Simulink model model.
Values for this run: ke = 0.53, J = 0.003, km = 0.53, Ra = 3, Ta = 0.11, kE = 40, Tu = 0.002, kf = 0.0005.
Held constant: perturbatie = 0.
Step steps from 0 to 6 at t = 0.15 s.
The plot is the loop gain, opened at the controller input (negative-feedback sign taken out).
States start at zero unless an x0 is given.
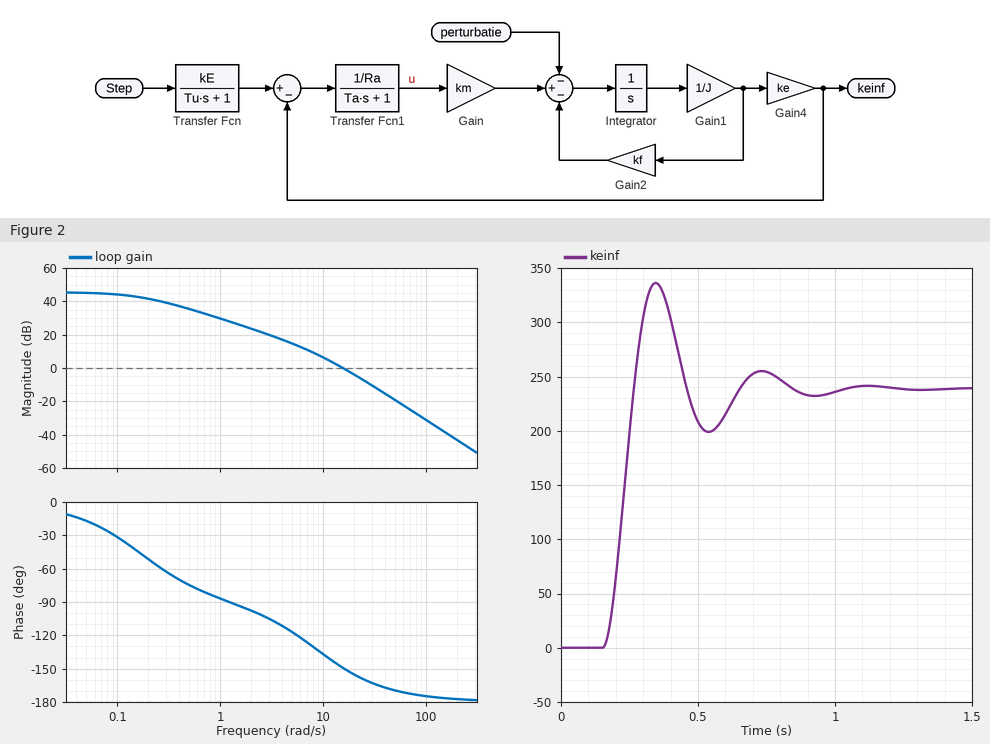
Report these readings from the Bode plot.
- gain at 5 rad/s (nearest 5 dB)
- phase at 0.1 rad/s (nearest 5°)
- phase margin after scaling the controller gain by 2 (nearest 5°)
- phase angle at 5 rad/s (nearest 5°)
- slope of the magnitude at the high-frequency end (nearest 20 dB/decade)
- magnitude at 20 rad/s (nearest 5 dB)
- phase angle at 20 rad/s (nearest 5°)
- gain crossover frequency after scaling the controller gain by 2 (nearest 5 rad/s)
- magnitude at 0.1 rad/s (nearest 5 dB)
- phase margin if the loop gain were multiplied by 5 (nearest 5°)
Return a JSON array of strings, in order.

["15 dB", "-30°", "20°", "-115°", "-40 dB/decade", "-5 dB", "-155°", "25 rad/s", "45 dB", "15°"]
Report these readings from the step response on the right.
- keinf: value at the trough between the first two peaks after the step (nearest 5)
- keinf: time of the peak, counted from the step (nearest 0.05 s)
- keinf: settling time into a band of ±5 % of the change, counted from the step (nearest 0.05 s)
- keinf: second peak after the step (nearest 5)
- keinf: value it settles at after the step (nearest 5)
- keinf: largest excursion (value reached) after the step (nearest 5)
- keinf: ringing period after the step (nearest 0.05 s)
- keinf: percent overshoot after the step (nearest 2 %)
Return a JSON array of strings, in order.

["200", "0.20 s", "0.65 s", "255", "240", "335", "0.40 s", "40 %"]
